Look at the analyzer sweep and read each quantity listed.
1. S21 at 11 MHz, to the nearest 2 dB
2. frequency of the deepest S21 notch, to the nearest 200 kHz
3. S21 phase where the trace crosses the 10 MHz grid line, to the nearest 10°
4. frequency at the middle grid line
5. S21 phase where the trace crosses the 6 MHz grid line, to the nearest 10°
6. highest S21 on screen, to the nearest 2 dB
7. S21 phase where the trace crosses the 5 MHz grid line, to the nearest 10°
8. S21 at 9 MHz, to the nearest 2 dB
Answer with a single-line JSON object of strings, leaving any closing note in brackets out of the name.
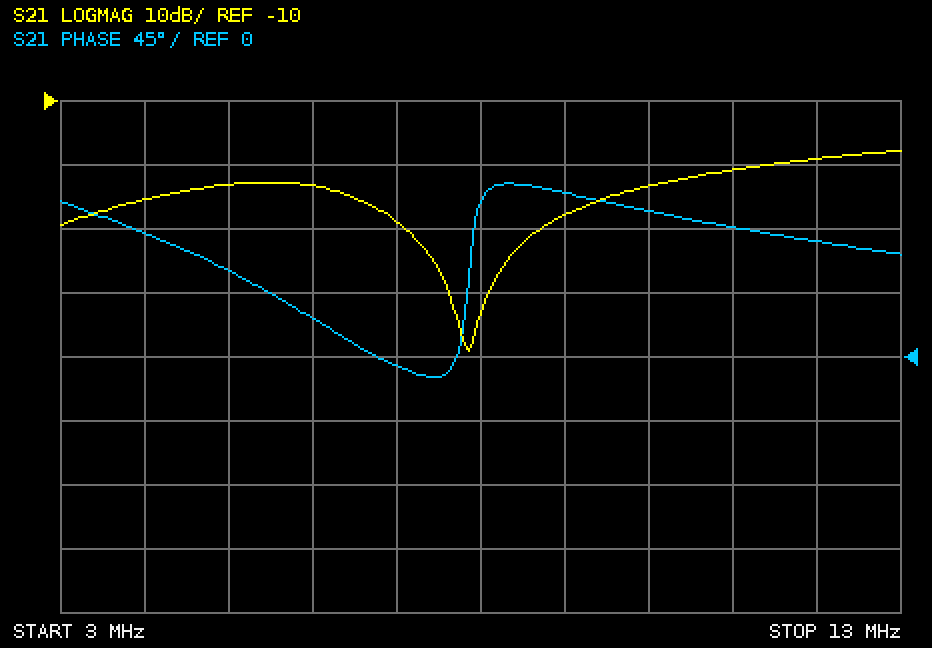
{"S21 at 11 MHz, to the nearest 2 dB": "-20 dB", "frequency of the deepest S21 notch, to the nearest 200 kHz": "7.8 MHz", "S21 phase where the trace crosses the 10 MHz grid line, to the nearest 10°": "100°", "frequency at the middle grid line": "8 MHz", "S21 phase where the trace crosses the 6 MHz grid line, to the nearest 10°": "30°", "highest S21 on screen, to the nearest 2 dB": "-18 dB", "S21 phase where the trace crosses the 5 MHz grid line, to the nearest 10°": "60°", "S21 at 9 MHz, to the nearest 2 dB": "-28 dB"}
